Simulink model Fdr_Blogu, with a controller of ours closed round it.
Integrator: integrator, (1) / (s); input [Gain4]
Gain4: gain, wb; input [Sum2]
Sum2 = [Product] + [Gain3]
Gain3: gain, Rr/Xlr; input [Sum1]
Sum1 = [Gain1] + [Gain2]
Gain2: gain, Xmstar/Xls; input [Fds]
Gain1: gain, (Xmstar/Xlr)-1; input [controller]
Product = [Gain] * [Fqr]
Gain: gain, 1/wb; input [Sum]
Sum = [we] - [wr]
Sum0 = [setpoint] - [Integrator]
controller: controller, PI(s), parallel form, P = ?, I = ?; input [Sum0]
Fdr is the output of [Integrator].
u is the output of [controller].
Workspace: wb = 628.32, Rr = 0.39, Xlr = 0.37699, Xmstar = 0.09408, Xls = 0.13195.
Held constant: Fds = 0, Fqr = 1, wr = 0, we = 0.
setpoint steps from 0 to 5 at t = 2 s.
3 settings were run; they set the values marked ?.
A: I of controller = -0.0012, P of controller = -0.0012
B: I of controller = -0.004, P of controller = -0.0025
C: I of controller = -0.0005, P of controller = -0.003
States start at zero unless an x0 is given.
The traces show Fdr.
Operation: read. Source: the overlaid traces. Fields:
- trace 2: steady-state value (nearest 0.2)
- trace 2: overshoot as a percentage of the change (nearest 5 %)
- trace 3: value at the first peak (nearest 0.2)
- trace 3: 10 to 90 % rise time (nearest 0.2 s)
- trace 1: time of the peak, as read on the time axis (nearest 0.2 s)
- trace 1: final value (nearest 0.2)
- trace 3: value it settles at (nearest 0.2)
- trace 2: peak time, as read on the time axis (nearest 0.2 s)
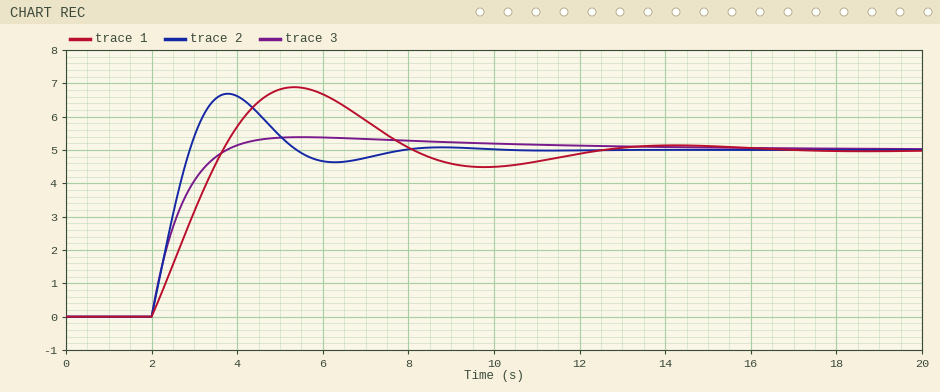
5.0
35 %
5.4
1.2 s
5.4 s
5.0
5.0
3.8 s
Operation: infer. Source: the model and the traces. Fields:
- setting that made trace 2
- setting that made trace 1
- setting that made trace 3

B
A
C
